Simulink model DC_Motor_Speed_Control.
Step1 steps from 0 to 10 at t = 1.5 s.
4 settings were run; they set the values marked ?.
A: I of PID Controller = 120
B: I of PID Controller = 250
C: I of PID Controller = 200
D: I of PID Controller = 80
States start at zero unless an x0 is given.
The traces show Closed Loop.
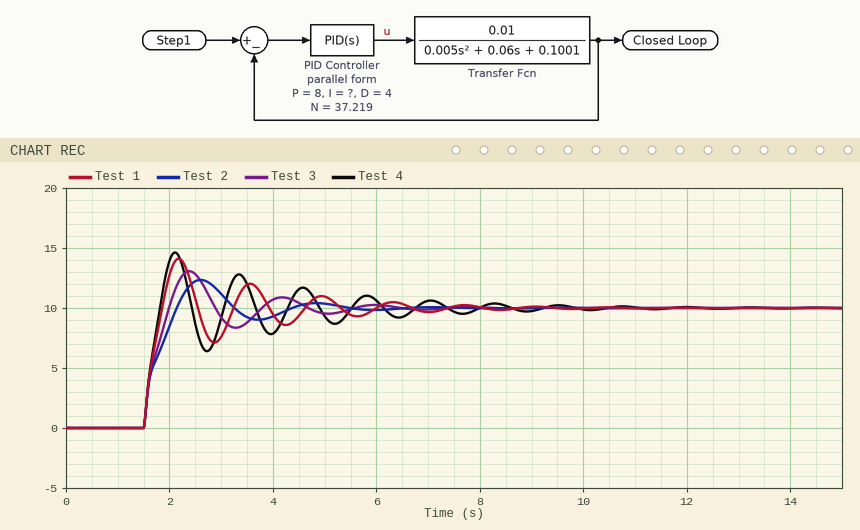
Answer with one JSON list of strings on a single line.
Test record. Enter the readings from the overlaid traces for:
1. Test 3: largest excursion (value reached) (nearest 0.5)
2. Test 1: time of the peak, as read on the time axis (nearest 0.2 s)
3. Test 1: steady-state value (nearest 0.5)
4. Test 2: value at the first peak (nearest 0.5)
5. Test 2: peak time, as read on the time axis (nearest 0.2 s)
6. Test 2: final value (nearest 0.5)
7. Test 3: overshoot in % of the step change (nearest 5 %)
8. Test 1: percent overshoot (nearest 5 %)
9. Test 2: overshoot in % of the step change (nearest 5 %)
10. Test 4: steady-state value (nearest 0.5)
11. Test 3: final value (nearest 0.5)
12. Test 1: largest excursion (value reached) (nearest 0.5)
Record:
["13.0", "2.2 s", "10.0", "12.5", "2.6 s", "10.0", "30 %", "40 %", "25 %", "10.0", "10.0", "14.0"]
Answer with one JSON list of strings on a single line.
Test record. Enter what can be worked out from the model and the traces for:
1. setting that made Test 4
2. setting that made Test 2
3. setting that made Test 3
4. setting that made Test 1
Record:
["B", "D", "A", "C"]
